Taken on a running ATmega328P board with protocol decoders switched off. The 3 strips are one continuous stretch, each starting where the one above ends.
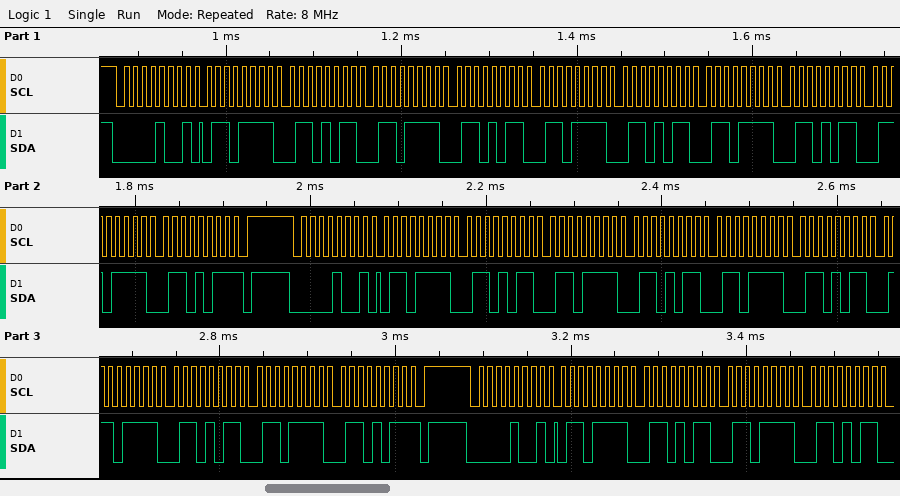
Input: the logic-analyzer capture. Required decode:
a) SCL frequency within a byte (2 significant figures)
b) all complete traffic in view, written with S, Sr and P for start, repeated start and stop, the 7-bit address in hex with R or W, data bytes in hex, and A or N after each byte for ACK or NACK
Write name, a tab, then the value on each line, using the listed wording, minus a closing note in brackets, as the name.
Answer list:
SCL frequency within a byte	100 kHz
all complete traffic in view, written with S, Sr and P for start, repeated start and stop, the 7-bit address in hex with R or W, data bytes in hex, and A or N after each byte for ACK or NACK	S 04R A 6F A 6B A 6F A 6B A 6F A 6B A 6F A 6B A 6F A 6B N P S 04R A 6F A 6B A 6F A 6B A 6F A 6B A 6F A 6B A 6F A 6B N P S 04R A 6F A 6B A 6F A 6B A
